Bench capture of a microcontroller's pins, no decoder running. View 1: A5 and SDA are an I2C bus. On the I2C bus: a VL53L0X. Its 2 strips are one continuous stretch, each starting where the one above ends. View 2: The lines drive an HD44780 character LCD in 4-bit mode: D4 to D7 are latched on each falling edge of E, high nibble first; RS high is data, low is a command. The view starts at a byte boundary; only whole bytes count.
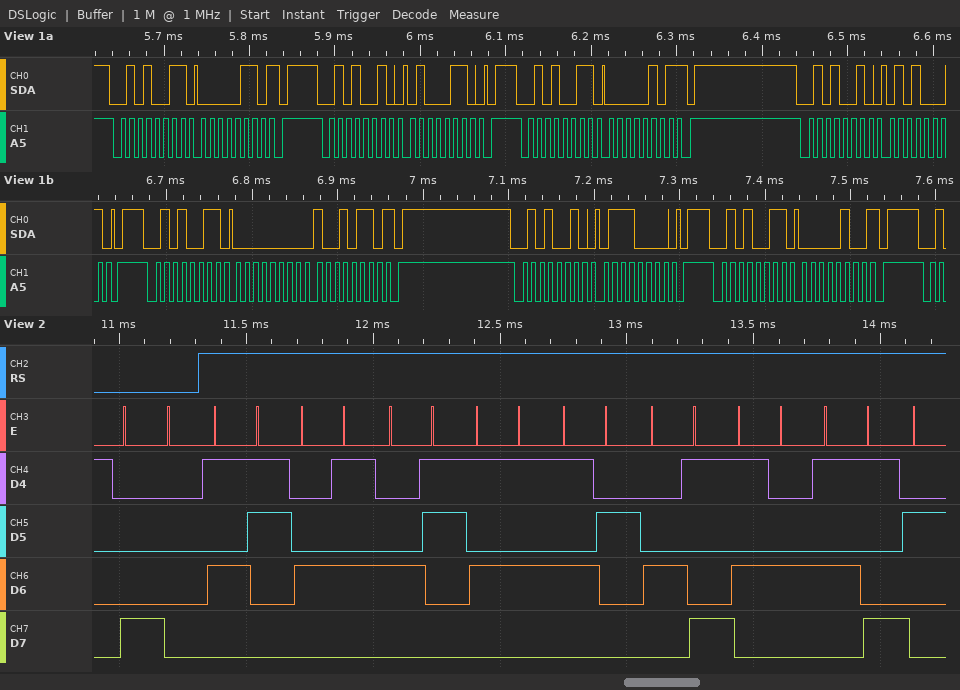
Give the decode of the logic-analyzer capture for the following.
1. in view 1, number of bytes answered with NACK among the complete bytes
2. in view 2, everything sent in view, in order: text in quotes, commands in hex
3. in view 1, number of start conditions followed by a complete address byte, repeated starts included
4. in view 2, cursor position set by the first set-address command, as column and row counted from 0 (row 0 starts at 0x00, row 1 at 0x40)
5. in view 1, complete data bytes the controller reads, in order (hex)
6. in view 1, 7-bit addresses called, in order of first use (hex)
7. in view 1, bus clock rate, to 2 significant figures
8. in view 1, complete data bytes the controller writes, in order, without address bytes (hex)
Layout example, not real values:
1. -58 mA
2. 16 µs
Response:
1. 4
2. 0x80 "SECURITY"
3. 7
4. column 0, row 0
5. 06 05 00 96 04
6. 0x29
7. 100 kHz
8. 46 51 70
